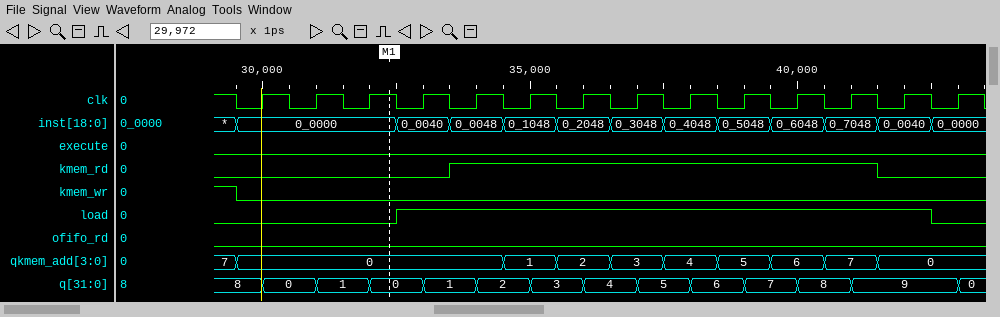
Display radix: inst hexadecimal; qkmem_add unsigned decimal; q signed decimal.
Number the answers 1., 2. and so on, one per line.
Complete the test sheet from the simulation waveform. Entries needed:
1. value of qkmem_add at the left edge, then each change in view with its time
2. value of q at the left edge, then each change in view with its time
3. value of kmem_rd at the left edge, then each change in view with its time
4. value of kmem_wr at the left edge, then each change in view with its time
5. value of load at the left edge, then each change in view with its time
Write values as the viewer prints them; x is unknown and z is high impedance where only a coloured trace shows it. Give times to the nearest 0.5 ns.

1. 7, 0 at 29.5 ns, 1 at 34.5 ns, 2 at 35.5 ns, 3 at 36.5 ns, 4 at 37.5 ns, 5 at 38.5 ns, 6 at 39.5 ns, 7 at 40.5 ns, 0 at 41.5 ns
2. 8, 0 at 30 ns, 1 at 31 ns, 0 at 32 ns, 1 at 33 ns, 2 at 34 ns, 3 at 35 ns, 4 at 36 ns, 5 at 37 ns, 6 at 38 ns, 7 at 39 ns, 8 at 40 ns, 9 at 41 ns, 0 at 43 ns
3. 0, 1 at 33.5 ns, 0 at 41.5 ns
4. 1, 0 at 29.5 ns
5. 0, 1 at 32.5 ns, 0 at 42.5 ns
